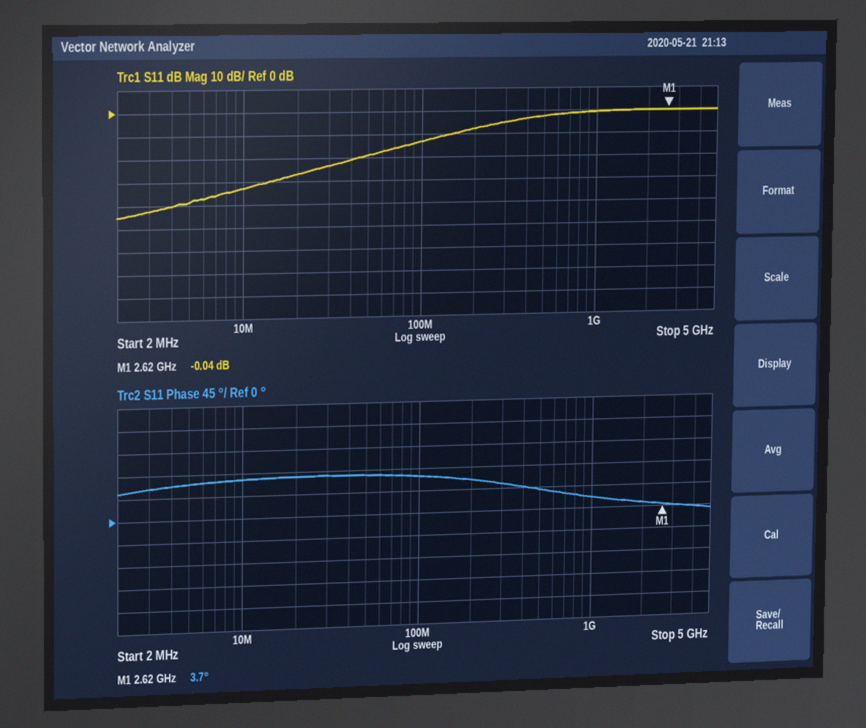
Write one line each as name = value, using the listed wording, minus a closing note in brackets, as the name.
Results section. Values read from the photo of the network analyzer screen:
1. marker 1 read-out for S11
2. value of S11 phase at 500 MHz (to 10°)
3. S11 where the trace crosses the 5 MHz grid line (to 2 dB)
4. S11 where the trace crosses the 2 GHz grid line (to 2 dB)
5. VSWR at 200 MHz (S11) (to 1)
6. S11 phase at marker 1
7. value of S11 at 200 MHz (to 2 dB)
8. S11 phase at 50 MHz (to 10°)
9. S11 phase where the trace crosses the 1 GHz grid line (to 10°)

marker 1 read-out for S11 = -0.04 dB
value of S11 phase at 500 MHz = 40°
S11 where the trace crosses the 5 MHz grid line = -38 dB
S11 where the trace crosses the 2 GHz grid line = 0 dB
VSWR at 200 MHz (S11) = 2
S11 phase at marker 1 = 3.7°
value of S11 at 200 MHz = -8 dB
S11 phase at 50 MHz = 80°
S11 phase where the trace crosses the 1 GHz grid line = 20°
